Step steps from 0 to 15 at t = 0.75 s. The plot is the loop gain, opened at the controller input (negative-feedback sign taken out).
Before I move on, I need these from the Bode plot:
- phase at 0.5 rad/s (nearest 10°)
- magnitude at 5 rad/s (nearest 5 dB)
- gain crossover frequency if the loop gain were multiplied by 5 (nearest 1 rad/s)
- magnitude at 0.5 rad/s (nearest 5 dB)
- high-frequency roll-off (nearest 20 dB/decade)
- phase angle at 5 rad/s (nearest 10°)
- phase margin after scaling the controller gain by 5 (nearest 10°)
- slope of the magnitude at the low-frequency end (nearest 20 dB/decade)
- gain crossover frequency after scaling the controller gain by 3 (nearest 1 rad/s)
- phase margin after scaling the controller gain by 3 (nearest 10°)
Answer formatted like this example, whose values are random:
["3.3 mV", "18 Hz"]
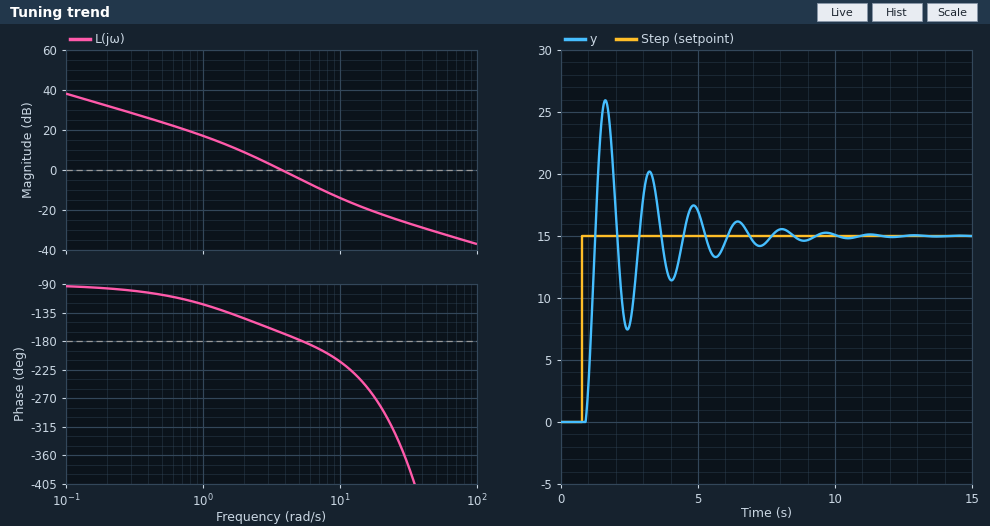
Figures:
["-110°", "-5 dB", "10 rad/s", "25 dB", "-20 dB/decade", "-180°", "-30°", "-20 dB/decade", "7 rad/s", "-10°"]
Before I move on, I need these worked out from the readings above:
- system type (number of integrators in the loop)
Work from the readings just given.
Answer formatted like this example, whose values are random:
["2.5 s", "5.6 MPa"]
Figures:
["1"]
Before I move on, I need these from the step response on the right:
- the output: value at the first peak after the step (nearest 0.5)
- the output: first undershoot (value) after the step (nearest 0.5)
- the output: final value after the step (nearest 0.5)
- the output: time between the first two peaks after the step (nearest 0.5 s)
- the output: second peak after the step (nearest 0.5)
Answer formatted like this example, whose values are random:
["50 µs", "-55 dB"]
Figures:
["26.0", "7.5", "15.0", "1.5 s", "20.0"]
